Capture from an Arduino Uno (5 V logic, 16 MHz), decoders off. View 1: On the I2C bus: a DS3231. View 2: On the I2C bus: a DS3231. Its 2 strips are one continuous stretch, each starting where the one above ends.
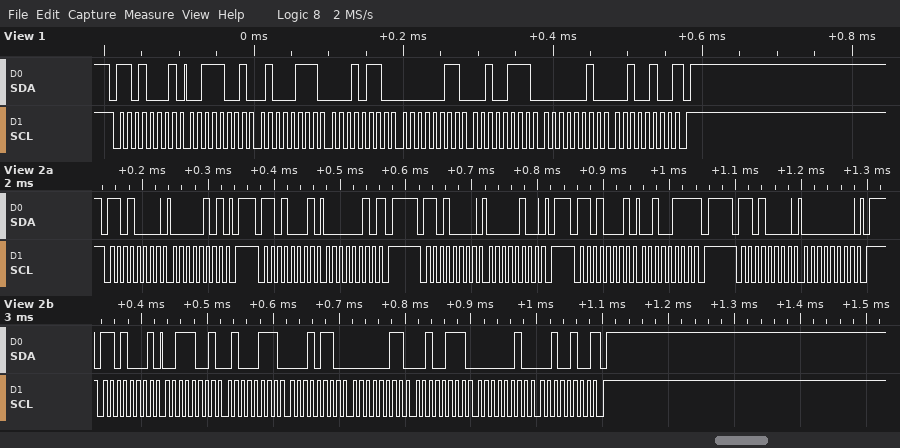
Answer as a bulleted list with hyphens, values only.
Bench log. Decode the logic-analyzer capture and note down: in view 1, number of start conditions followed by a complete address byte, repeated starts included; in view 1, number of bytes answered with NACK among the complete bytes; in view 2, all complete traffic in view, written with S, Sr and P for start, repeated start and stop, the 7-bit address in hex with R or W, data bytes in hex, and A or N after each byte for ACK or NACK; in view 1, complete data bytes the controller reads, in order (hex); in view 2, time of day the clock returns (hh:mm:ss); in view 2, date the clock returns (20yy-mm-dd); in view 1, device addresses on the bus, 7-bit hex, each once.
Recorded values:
- 1
- 1
- S 68W A 05 A P S 68R A 02 N P S 68W A 04 A P S 68R A 27 N P S 68W A 00 A P S 68R A 39 A 47 A 16 A 03 A 27 A 02 A 24 N P
- 39 47 16 03 27 02 24
- 16:47:39
- 2024-02-27
- 0x68
